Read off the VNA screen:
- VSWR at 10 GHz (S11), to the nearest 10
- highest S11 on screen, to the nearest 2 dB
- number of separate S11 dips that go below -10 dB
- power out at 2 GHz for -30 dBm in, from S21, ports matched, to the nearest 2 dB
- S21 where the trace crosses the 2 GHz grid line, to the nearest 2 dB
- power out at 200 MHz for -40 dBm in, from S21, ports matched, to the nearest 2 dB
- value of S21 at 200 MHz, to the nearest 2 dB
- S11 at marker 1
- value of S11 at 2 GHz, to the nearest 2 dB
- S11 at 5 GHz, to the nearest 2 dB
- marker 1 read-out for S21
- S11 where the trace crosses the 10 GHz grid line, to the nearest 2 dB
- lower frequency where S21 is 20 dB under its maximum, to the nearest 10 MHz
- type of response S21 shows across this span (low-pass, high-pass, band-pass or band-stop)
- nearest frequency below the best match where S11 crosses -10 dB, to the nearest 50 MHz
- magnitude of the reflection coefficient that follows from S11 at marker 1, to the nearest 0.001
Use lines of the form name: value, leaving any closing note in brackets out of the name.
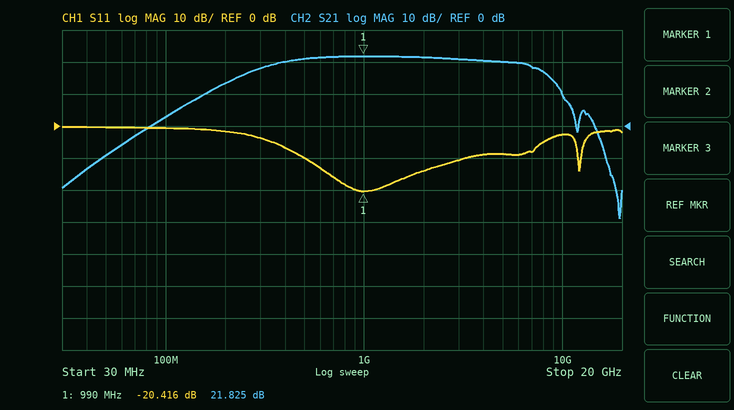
VSWR at 10 GHz (S11), to the nearest 10: 10
highest S11 on screen, to the nearest 2 dB: 0 dB
number of separate S11 dips that go below -10 dB: 2
power out at 2 GHz for -30 dBm in, from S21, ports matched, to the nearest 2 dB: -8 dBm
S21 where the trace crosses the 2 GHz grid line, to the nearest 2 dB: 22 dB
power out at 200 MHz for -40 dBm in, from S21, ports matched, to the nearest 2 dB: -26 dBm
value of S21 at 200 MHz, to the nearest 2 dB: 14 dB
S11 at marker 1: -20.416 dB
value of S11 at 2 GHz, to the nearest 2 dB: -14 dB
S11 at 5 GHz, to the nearest 2 dB: -8 dB
marker 1 read-out for S21: 21.825 dB
S11 where the trace crosses the 10 GHz grid line, to the nearest 2 dB: -2 dB
lower frequency where S21 is 20 dB under its maximum, to the nearest 10 MHz: 90 MHz
type of response S21 shows across this span: band-pass
nearest frequency below the best match where S11 crosses -10 dB, to the nearest 50 MHz: 500 MHz
magnitude of the reflection coefficient that follows from S11 at marker 1, to the nearest 0.001: 0.095
